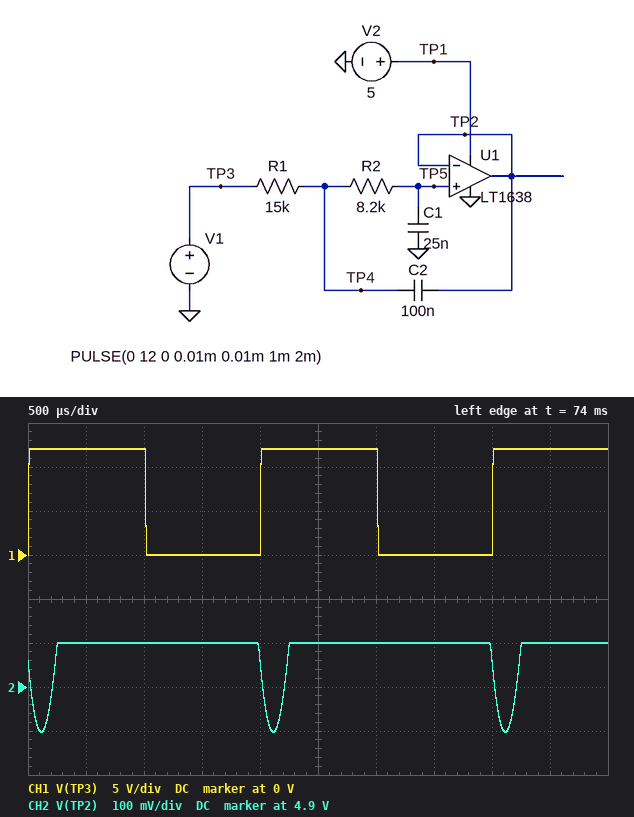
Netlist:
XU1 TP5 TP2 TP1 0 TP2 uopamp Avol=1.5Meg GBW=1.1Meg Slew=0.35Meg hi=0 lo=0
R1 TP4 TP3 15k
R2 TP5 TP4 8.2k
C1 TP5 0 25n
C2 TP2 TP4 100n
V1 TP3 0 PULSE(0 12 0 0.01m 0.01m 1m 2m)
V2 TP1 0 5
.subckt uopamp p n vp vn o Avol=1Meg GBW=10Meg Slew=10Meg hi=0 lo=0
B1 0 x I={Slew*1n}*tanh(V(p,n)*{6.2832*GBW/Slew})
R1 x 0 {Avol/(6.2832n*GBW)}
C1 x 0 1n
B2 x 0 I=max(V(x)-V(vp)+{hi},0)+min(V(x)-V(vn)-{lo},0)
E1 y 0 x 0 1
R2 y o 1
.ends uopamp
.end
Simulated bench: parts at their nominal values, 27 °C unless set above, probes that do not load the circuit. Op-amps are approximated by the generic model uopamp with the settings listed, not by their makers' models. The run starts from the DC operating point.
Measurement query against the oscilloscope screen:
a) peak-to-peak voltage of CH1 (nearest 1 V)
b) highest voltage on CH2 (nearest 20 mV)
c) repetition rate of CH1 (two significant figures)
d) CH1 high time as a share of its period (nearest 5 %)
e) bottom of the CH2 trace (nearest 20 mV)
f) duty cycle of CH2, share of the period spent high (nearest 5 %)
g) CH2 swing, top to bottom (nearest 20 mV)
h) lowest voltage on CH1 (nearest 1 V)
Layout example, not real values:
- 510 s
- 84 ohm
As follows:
- 12 V
- 5.00 V
- 500 Hz
- 50 %
- 4.80 V
- 90 %
- 200 mV
- 0 V
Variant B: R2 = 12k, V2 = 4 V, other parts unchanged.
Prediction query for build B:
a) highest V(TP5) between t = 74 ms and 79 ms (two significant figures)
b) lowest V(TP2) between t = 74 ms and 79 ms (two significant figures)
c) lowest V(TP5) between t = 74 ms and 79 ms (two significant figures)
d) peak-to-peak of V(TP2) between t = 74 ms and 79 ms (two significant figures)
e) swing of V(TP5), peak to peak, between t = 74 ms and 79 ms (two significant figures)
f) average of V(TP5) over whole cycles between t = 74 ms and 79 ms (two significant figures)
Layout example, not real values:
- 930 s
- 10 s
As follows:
- 7.1 V
- 4.0 V
- 5.0 V
- 1.1 mV
- 2.1 V
- 6.1 V
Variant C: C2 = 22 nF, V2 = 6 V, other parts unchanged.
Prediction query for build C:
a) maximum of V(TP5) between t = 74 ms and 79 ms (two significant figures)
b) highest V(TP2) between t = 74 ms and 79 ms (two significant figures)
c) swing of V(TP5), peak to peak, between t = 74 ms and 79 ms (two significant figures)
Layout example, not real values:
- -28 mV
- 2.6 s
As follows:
- 9.4 V
- 6.0 V
- 7.2 V
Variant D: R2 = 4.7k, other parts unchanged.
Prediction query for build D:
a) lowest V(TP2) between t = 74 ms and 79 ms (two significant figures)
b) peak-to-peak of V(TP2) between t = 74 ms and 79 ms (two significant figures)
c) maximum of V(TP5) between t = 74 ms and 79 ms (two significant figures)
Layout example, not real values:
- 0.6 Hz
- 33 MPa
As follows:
- 4.5 V
- 490 mV
- 7.5 V
